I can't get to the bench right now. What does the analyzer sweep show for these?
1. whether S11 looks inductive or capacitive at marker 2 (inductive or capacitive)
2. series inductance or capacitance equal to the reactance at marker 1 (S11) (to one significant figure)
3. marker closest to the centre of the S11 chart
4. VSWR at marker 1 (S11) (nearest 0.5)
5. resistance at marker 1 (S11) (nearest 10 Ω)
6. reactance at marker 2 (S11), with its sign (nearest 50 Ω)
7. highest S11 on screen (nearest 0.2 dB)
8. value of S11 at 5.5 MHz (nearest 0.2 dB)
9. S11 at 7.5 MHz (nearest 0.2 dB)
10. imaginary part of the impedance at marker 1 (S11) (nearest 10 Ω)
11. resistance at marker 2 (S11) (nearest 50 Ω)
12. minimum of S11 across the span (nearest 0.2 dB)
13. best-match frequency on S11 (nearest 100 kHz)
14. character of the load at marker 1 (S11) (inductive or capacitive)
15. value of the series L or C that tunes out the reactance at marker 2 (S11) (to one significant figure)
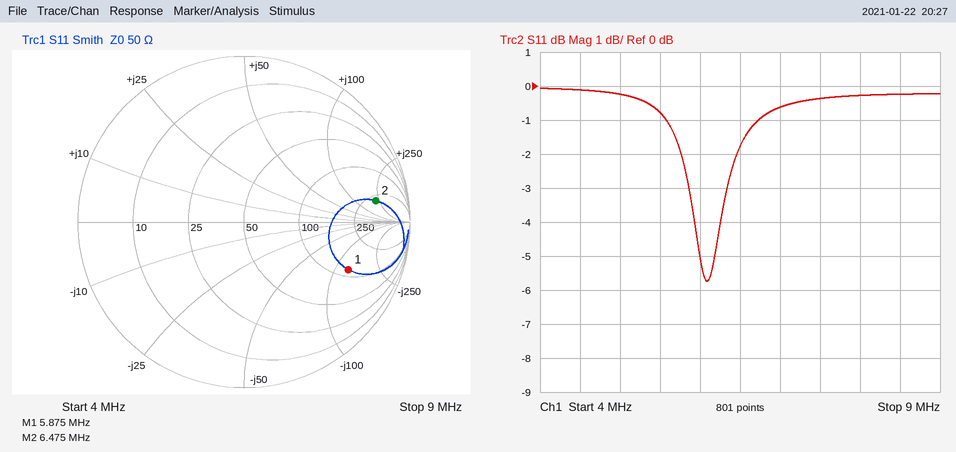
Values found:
inductive
200 pF
marker 1
5.5
120 Ω
+200 Ω
0.0 dB
-0.8 dB
-0.4 dB
-130 Ω
300 Ω
-5.8 dB
6.1 MHz
capacitive
100 pF
